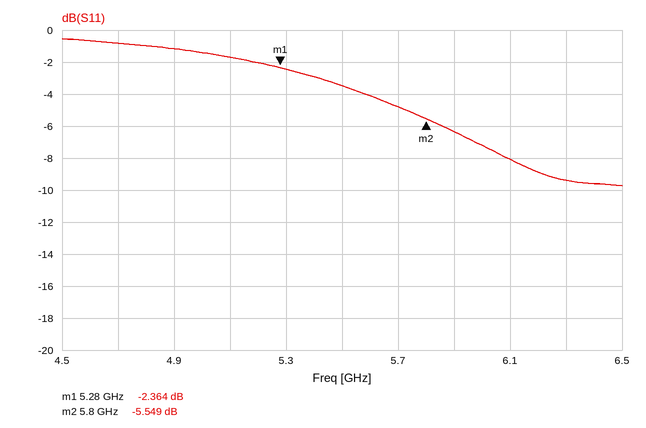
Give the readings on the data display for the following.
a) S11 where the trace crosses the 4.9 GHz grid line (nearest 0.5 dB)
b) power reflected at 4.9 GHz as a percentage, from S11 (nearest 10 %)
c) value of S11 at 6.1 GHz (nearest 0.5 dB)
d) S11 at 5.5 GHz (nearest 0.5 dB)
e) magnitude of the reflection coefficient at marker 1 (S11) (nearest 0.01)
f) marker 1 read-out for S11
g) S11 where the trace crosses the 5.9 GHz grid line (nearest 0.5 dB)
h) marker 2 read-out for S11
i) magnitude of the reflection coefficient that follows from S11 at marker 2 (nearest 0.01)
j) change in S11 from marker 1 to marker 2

-1.0 dB
80 %
-8.0 dB
-3.5 dB
0.76
-2.364 dB
-6.5 dB
-5.549 dB
0.53
-3.185 dB
